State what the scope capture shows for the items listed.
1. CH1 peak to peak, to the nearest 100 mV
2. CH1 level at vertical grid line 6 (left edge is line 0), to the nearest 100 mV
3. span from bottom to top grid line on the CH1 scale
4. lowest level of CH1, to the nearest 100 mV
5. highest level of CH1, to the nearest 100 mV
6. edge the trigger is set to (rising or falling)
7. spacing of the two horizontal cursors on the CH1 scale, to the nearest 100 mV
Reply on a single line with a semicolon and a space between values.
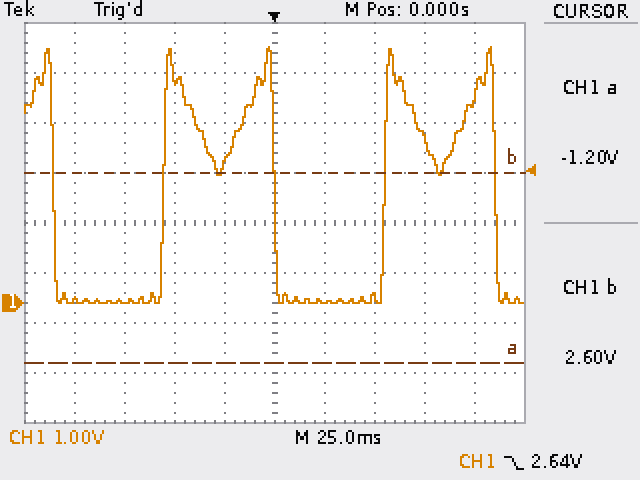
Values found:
5.1 V; 0.0 V; 8 V; 0.0 V; 5.1 V; falling; 3.8 V
